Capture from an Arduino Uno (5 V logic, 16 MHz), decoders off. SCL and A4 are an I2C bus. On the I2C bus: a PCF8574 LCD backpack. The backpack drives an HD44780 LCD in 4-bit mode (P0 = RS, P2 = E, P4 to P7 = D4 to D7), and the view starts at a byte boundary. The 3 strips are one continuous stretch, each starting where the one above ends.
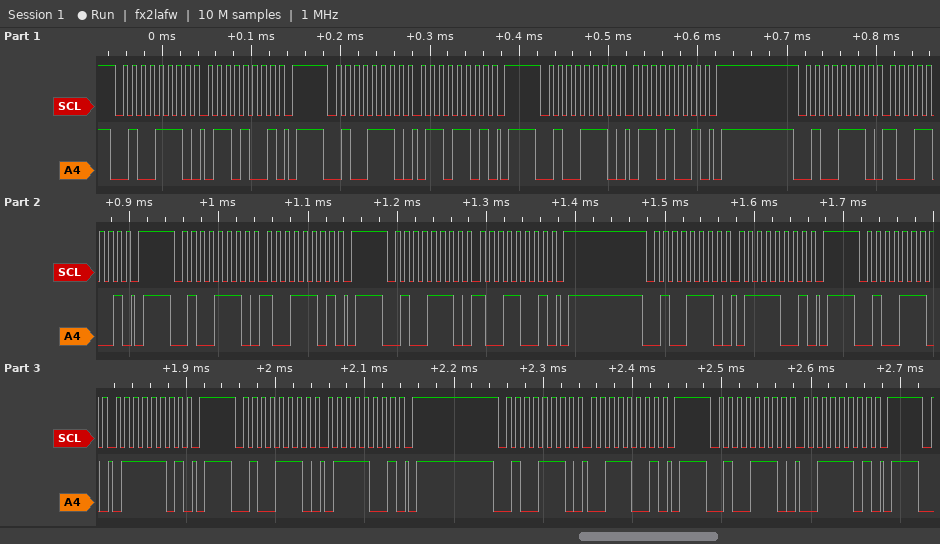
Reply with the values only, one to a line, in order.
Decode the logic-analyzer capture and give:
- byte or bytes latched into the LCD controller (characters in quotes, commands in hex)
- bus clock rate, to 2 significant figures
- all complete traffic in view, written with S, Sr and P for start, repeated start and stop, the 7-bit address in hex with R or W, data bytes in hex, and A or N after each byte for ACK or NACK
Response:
'i'
100 kHz
S 27W A 69 A P S 27W A 6D A P S 27W A 69 A P S 27W A 99 A P S 27W A 9D A P S 27W A 99 A P S 27W A 79 A P S 27W A 7D A P S 27W A 79 A P S 27W A 39 A P S 27W A 3D A P
